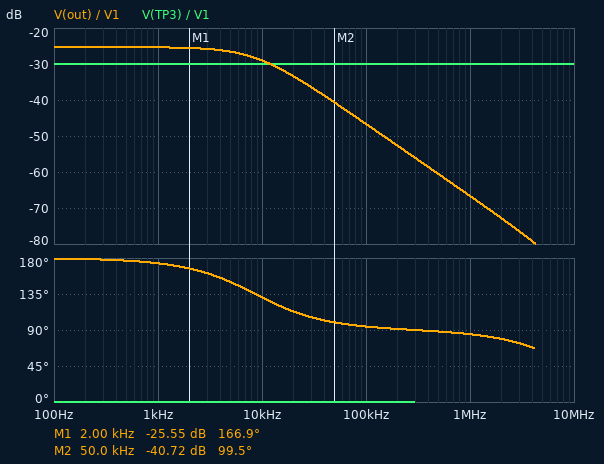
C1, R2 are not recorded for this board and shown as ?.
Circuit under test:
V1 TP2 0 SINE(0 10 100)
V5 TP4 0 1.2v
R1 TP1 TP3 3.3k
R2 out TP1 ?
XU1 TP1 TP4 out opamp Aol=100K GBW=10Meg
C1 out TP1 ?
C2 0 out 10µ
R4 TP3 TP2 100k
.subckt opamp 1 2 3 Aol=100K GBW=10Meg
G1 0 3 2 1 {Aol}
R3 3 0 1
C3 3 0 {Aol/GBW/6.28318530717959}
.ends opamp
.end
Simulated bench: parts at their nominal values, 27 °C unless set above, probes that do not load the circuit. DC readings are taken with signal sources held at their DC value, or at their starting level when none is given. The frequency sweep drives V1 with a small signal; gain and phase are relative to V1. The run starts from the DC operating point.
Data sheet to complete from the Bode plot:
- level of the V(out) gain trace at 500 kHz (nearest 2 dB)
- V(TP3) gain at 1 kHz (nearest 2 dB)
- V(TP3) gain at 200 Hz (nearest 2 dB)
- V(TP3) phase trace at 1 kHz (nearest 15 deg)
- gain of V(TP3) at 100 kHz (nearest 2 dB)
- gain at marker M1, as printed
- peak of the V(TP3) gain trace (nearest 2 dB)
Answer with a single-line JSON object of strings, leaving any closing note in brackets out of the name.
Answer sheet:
{"level of the V(out) gain trace at 500 kHz": "-60 dB", "V(TP3) gain at 1 kHz": "-30 dB", "V(TP3) gain at 200 Hz": "-30 dB", "V(TP3) phase trace at 1 kHz": "0 deg", "gain of V(TP3) at 100 kHz": "-30 dB", "gain at marker M1, as printed": "-25.55 dB", "peak of the V(TP3) gain trace": "-30 dB"}
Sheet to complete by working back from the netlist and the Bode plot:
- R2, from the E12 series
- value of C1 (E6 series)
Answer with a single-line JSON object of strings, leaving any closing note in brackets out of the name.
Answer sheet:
{"R2, from the E12 series": "5.6 kΩ", "value of C1": "3.3 nF"}
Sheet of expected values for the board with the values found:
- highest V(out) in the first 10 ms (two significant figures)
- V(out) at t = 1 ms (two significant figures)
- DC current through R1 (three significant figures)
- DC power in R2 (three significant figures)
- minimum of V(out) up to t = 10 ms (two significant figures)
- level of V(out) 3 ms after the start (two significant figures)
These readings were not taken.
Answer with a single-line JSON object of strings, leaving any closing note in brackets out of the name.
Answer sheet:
{"highest V(out) in the first 10 ms": "1.8 V", "V(out) at t = 1 ms": "950 mV", "DC current through R1": "11.6 µA", "DC power in R2": "756 nW", "minimum of V(out) up to t = 10 ms": "720 mV", "level of V(out) 3 ms after the start": "750 mV"}
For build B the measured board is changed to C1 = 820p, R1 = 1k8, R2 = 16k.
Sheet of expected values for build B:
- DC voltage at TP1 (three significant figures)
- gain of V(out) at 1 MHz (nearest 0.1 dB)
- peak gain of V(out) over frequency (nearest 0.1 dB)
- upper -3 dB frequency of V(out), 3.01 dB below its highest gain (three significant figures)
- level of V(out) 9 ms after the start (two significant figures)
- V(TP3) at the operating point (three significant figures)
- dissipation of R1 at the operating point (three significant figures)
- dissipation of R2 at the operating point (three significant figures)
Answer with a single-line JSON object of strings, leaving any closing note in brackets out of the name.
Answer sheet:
{"DC voltage at TP1": "1.20 V", "gain of V(out) at 1 MHz": "-54.4 dB", "peak gain of V(out) over frequency": "-16.1 dB", "upper -3 dB frequency of V(out), 3.01 dB below its highest gain": "12.1 kHz", "level of V(out) 9 ms after the start": "2.3 V", "V(TP3) at the operating point": "1.18 V", "dissipation of R1 at the operating point": "250 nW", "dissipation of R2 at the operating point": "2.22 µW"}
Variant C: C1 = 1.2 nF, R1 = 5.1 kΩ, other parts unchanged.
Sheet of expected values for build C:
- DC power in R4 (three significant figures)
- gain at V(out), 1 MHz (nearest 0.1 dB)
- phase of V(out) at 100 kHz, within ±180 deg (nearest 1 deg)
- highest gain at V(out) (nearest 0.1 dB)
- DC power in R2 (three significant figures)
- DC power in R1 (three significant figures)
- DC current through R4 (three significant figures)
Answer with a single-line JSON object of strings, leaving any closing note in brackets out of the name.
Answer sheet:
{"DC power in R4": "13.0 µW", "gain at V(out), 1 MHz": "-58.0 dB", "phase of V(out) at 100 kHz, within ±180 deg": "103 deg", "highest gain at V(out)": "-25.5 dB", "DC power in R2": "730 nW", "DC power in R1": "665 nW", "DC current through R4": "11.4 µA"}
